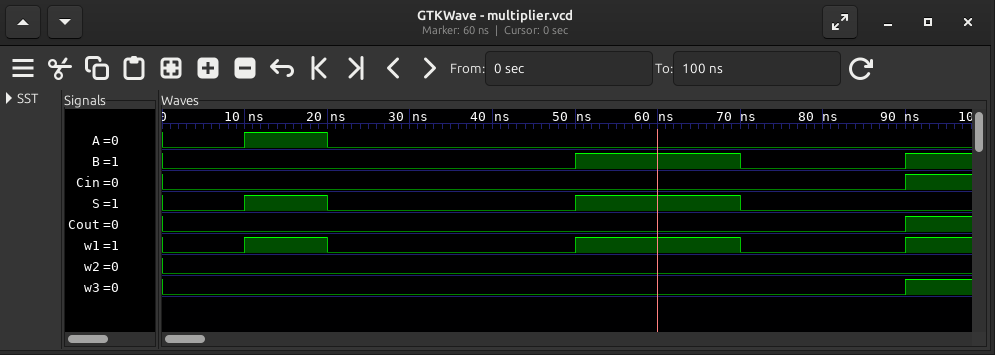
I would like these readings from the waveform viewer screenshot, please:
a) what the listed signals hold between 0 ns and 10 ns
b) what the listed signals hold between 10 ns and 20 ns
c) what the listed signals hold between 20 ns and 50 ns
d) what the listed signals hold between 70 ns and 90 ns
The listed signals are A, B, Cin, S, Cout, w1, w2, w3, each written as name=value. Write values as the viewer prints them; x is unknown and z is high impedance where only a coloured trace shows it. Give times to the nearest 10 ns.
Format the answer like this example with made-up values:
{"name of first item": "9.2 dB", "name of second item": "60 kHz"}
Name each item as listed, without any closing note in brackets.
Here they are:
{"what the listed signals hold between 0 ns and 10 ns": "A=0, B=0, Cin=0, S=0, Cout=0, w1=0, w2=0, w3=0", "what the listed signals hold between 10 ns and 20 ns": "A=1, B=0, Cin=0, S=1, Cout=0, w1=1, w2=0, w3=0", "what the listed signals hold between 20 ns and 50 ns": "A=0, B=0, Cin=0, S=0, Cout=0, w1=0, w2=0, w3=0", "what the listed signals hold between 70 ns and 90 ns": "A=0, B=0, Cin=0, S=0, Cout=0, w1=0, w2=0, w3=0"}
